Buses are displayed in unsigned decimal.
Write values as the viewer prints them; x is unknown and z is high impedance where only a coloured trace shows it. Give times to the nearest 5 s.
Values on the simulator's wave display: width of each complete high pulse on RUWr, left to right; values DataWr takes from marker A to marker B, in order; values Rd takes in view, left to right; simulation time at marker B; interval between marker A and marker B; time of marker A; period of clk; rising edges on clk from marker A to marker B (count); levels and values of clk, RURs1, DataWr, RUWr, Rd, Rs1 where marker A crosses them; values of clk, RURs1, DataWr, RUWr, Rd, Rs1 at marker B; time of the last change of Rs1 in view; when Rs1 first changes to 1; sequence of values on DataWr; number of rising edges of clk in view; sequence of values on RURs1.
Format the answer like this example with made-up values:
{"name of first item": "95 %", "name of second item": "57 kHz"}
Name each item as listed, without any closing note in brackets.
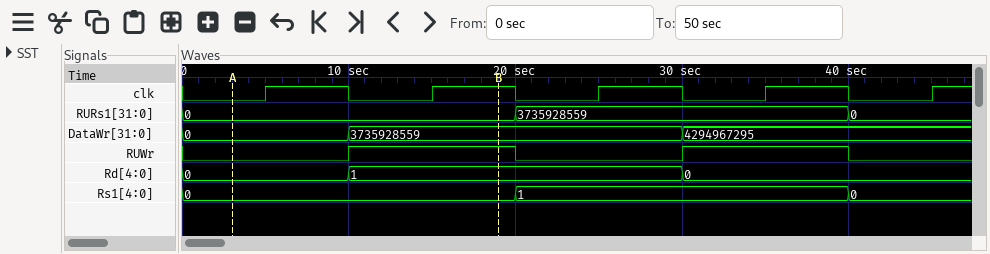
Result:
{"width of each complete high pulse on RUWr, left to right": "10 s, 10 s", "values DataWr takes from marker A to marker B, in order": "0, 3735928559", "values Rd takes in view, left to right": "0, 1, 0", "simulation time at marker B": "20 s", "interval between marker A and marker B": "15 s", "time of marker A": "5 s", "period of clk": "10 s", "rising edges on clk from marker A to marker B": "2", "levels and values of clk, RURs1, DataWr, RUWr, Rd, Rs1 where marker A crosses them": "clk=0, RURs1=0, DataWr=0, RUWr=0, Rd=0, Rs1=0", "values of clk, RURs1, DataWr, RUWr, Rd, Rs1 at marker B": "clk=1, RURs1=0, DataWr=3735928559, RUWr=1, Rd=1, Rs1=0", "time of the last change of Rs1 in view": "40 s", "when Rs1 first changes to 1": "20 s", "sequence of values on DataWr": "0, 3735928559, 4294967295", "number of rising edges of clk in view": "5", "sequence of values on RURs1": "0, 3735928559, 0"}
